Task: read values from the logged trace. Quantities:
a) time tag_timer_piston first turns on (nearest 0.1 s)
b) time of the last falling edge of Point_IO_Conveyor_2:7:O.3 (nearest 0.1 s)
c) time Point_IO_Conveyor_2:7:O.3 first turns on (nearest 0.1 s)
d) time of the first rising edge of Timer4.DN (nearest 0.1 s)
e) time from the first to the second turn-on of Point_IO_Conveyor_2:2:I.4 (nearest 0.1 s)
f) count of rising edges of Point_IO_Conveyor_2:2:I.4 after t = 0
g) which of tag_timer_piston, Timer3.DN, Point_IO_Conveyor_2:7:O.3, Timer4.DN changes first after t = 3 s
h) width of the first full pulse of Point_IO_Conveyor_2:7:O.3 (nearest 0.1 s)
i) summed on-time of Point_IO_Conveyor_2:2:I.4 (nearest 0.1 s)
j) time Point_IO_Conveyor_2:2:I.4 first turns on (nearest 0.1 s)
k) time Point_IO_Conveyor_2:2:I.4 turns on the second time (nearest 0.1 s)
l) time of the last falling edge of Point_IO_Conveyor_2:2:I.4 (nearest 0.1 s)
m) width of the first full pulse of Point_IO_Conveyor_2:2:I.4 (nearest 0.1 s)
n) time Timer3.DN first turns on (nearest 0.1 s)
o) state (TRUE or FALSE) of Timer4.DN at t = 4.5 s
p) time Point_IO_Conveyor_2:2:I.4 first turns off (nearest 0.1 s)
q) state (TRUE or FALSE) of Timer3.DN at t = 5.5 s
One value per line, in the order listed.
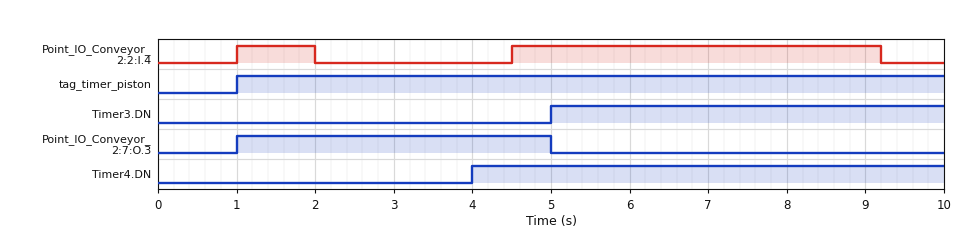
1.0 s
5.0 s
1.0 s
4.0 s
3.5 s
2
Timer4.DN
4.0 s
5.7 s
1.0 s
4.5 s
9.2 s
1.0 s
5.0 s
TRUE
2.0 s
TRUE
